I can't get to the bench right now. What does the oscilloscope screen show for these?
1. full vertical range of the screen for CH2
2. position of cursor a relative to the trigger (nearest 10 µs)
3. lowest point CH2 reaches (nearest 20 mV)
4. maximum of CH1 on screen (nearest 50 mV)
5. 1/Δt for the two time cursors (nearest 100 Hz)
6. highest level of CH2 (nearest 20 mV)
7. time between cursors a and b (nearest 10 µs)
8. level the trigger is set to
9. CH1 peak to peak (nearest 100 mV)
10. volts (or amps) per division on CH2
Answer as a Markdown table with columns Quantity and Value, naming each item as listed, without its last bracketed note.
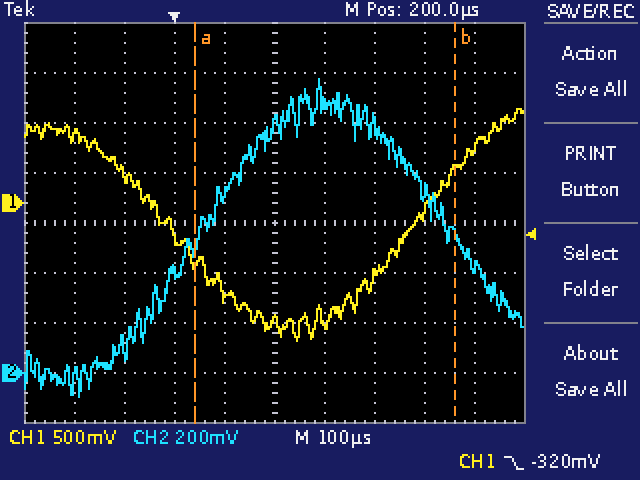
| Quantity | Value |
|---|---|
| full vertical range of the screen for CH2 | 1.6 V |
| position of cursor a relative to the trigger | +40 µs |
| lowest point CH2 reaches | -100 mV |
| maximum of CH1 on screen | 950 mV |
| 1/Δt for the two time cursors | 1.9 kHz |
| highest level of CH2 | 1.18 V |
| time between cursors a and b | 520 µs |
| level the trigger is set to | -320 mV |
| CH1 peak to peak | 2.30 V |
| volts (or amps) per division on CH2 | 200 mV |
